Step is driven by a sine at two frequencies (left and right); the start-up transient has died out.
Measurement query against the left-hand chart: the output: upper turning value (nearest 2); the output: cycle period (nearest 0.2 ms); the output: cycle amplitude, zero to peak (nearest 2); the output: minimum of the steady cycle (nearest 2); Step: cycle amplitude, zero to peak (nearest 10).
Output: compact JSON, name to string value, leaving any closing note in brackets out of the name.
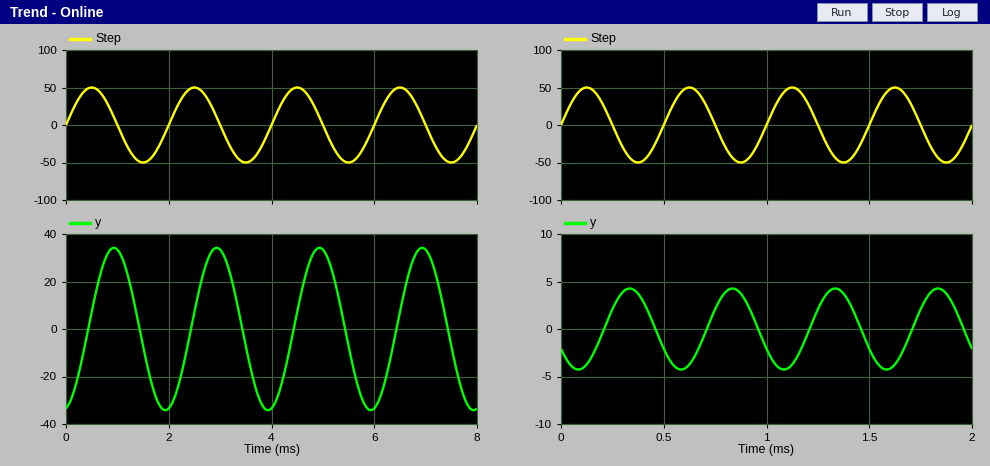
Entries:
{"the output: upper turning value": "34", "the output: cycle period": "2.0 ms", "the output: cycle amplitude, zero to peak": "34", "the output: minimum of the steady cycle": "-34", "Step: cycle amplitude, zero to peak": "50"}
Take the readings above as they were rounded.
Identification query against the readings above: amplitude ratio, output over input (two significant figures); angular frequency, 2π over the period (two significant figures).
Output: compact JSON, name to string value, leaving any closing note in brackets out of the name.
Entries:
{"amplitude ratio, output over input": "0.68", "angular frequency, 2π over the period": "3.1 rad/ms"}
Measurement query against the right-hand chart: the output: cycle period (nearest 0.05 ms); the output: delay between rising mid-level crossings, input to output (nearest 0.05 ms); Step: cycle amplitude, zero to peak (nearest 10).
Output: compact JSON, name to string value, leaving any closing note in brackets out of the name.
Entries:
{"the output: cycle period": "0.50 ms", "the output: delay between rising mid-level crossings, input to output": "0.20 ms", "Step: cycle amplitude, zero to peak": "50"}
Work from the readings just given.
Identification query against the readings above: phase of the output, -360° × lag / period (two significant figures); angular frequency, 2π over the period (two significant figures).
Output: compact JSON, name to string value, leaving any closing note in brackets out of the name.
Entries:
{"phase of the output, -360° × lag / period": "-140°", "angular frequency, 2π over the period": "13 rad/ms"}
